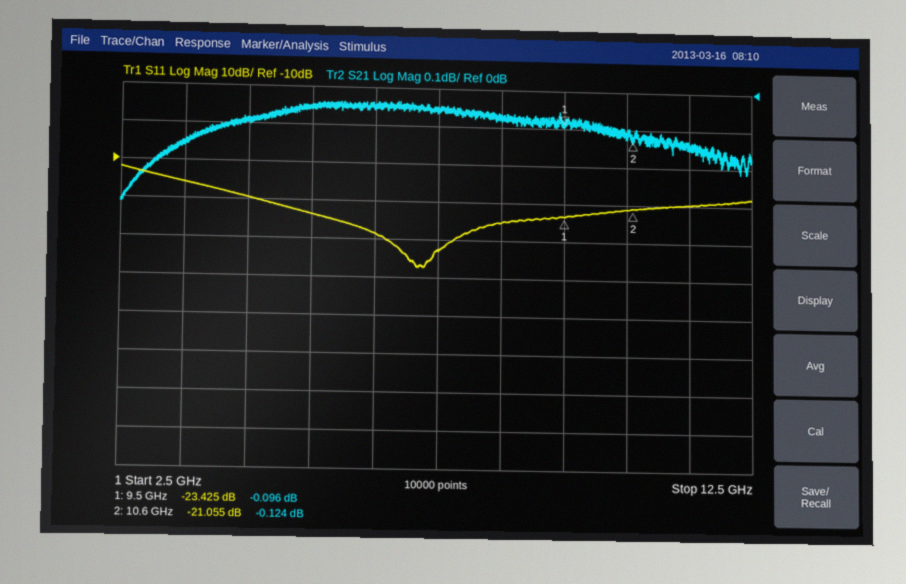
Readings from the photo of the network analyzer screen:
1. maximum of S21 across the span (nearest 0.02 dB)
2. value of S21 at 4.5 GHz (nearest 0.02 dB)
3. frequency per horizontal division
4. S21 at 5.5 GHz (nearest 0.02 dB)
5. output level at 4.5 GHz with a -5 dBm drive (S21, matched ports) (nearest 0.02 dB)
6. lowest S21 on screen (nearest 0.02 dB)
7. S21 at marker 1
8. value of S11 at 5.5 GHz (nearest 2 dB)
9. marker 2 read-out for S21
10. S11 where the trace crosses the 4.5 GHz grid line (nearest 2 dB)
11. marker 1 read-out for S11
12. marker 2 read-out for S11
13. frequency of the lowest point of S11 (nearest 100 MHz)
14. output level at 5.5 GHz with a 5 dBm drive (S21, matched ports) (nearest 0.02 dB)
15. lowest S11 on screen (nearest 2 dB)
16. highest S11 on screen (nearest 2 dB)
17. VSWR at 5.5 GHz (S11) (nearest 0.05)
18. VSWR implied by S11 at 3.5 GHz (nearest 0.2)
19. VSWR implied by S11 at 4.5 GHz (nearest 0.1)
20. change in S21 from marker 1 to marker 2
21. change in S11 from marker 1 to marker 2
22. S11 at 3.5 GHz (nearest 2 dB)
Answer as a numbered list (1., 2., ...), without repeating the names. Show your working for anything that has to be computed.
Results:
1. -0.04 dB
2. -0.10 dB
3. 1 GHz
4. -0.06 dB
5. -5 dBm + (-0.10 dB) = -5.10 dBm
6. -0.32 dB
7. -0.096 dB
8. -24 dB
9. -0.124 dB
10. -20 dB
11. -23.425 dB
12. -21.055 dB
13. 7.2 GHz
14. 5 dBm + (-0.06 dB) = 4.94 dBm
15. -38 dB
16. -12 dB
17. |Γ| = 10^(-24/20) = 0.0631; VSWR = (1 + 0.0631)/(1 − 0.0631) ≈ 1.13, so 1.15 to the nearest 0.05
18. |Γ| = 10^(-16/20) = 0.1585; VSWR = (1 + 0.1585)/(1 − 0.1585) ≈ 1.4
19. |Γ| = 10^(-20/20) = 0.1000; VSWR = (1 + 0.1000)/(1 − 0.1000) ≈ 1.2
20. -0.124 − (-0.096) = -0.028 dB
21. -21.055 − (-23.425) = 2.370 dB
22. -16 dB
